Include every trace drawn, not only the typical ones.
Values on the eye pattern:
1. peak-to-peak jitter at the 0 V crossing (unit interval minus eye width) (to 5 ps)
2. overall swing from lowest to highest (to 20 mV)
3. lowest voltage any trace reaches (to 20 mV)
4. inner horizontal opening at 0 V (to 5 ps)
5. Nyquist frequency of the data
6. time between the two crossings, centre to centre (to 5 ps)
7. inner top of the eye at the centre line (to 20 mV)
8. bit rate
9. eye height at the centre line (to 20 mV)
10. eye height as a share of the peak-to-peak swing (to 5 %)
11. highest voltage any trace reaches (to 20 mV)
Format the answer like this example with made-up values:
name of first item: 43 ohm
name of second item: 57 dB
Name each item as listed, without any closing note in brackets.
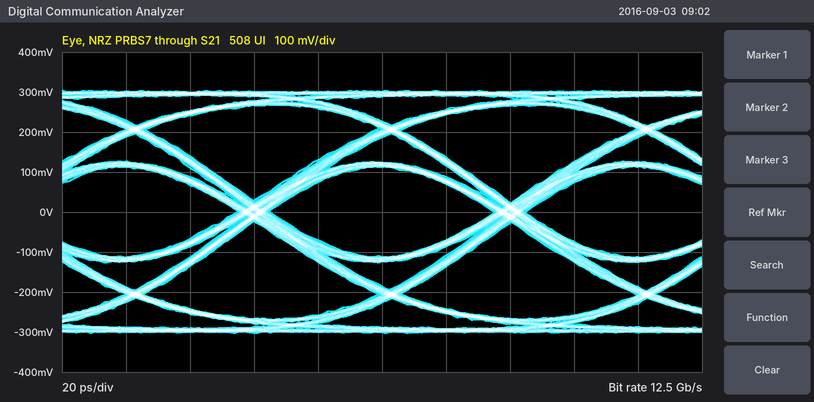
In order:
peak-to-peak jitter at the 0 V crossing (unit interval minus eye width): 10 ps
overall swing from lowest to highest: 600 mV
lowest voltage any trace reaches: -300 mV
inner horizontal opening at 0 V: 70 ps
Nyquist frequency of the data: 6.25 GHz
time between the two crossings, centre to centre: 80 ps
inner top of the eye at the centre line: 120 mV
bit rate: 12.5 Gb/s
eye height at the centre line: 220 mV
eye height as a share of the peak-to-peak swing: 35 %
highest voltage any trace reaches: 300 mV
